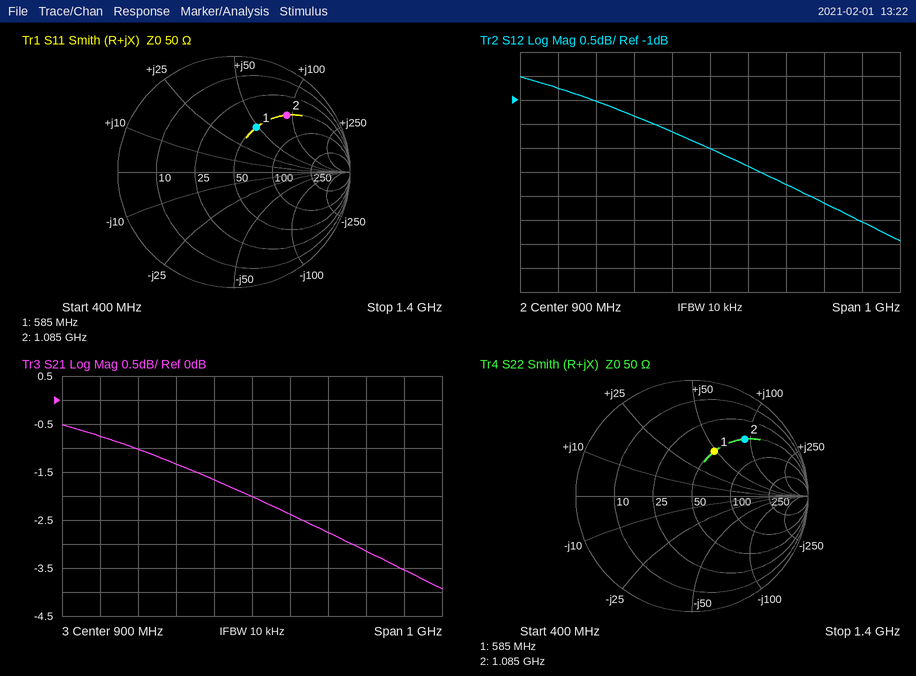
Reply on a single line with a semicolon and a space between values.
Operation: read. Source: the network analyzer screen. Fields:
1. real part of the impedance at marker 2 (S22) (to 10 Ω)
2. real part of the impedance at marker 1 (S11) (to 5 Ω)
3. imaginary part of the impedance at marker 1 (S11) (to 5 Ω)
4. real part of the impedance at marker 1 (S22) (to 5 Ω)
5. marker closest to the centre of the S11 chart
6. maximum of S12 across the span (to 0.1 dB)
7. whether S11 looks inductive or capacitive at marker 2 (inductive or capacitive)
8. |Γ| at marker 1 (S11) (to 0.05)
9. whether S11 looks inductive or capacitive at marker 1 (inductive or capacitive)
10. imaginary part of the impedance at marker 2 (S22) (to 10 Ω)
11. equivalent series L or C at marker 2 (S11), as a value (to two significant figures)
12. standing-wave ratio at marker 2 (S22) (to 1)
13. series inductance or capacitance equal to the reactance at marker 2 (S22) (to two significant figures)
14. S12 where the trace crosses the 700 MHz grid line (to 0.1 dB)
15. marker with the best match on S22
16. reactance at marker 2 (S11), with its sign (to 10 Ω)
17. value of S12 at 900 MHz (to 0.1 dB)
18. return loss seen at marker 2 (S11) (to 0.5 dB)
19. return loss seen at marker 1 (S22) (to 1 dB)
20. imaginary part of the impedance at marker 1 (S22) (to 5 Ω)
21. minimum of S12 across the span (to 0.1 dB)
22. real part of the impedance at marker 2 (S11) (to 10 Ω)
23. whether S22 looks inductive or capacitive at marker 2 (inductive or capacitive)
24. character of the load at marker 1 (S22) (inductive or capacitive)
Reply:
50 Ω; 50 Ω; +50 Ω; 50 Ω; marker 1; -0.5 dB; inductive; 0.45; inductive; +90 Ω; 13 nH; 5; 13 nH; -1.3 dB; marker 1; +90 Ω; -2.0 dB; 3.5 dB; 7 dB; +50 Ω; -3.9 dB; 50 Ω; inductive; inductive
